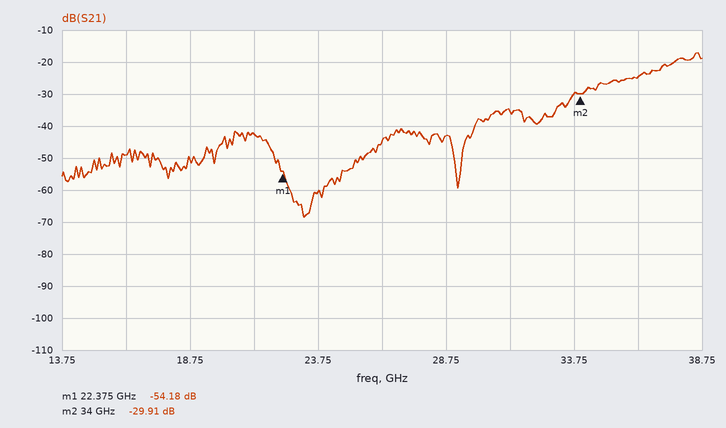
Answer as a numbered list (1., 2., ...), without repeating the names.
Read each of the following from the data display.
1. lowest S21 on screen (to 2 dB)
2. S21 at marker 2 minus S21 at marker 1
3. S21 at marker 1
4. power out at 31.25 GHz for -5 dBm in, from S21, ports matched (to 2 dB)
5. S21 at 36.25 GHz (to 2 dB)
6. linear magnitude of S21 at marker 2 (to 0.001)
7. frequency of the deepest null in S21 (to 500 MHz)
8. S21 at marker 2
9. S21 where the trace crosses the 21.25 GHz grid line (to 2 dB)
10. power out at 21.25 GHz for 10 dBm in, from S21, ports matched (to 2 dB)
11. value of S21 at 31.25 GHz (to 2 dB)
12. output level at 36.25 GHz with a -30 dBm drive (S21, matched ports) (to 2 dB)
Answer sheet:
1. -68 dB
2. 24.27 dB
3. -54.18 dB
4. -40 dBm
5. -24 dB
6. 0.032
7. 23.0 GHz
8. -29.91 dB
9. -42 dB
10. -32 dBm
11. -36 dB
12. -54 dBm
